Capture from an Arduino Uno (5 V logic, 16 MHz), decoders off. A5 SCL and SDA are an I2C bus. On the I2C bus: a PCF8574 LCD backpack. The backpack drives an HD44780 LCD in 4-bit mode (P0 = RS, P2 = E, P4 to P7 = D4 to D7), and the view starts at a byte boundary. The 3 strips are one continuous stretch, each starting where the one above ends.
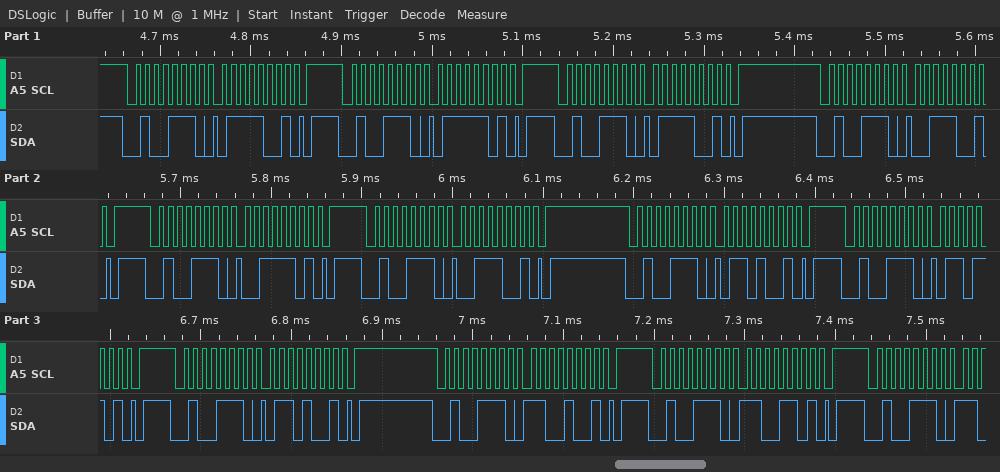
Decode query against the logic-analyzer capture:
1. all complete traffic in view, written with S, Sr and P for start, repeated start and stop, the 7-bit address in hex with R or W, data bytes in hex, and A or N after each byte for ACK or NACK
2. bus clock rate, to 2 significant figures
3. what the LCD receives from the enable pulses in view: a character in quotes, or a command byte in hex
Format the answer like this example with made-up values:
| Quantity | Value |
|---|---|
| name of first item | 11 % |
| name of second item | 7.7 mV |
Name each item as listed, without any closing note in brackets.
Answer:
| Quantity | Value |
|---|---|
| all complete traffic in view, written with S, Sr and P for start, repeated start and stop, the 7-bit address in hex with R or W, data bytes in hex, and A or N after each byte for ACK or NACK | S 27W A 79 A P S 27W A 7D A P S 27W A 79 A P S 27W A 39 A P S 27W A 3D A P S 27W A 39 A P S 27W A 69 A P S 27W A 6D A P S 27W A 69 A P S 27W A C9 A P S 27W A CD A P S 27W A |
| bus clock rate, to 2 significant figures | 100 kHz |
| what the LCD receives from the enable pulses in view: a character in quotes, or a command byte in hex | 's' |
